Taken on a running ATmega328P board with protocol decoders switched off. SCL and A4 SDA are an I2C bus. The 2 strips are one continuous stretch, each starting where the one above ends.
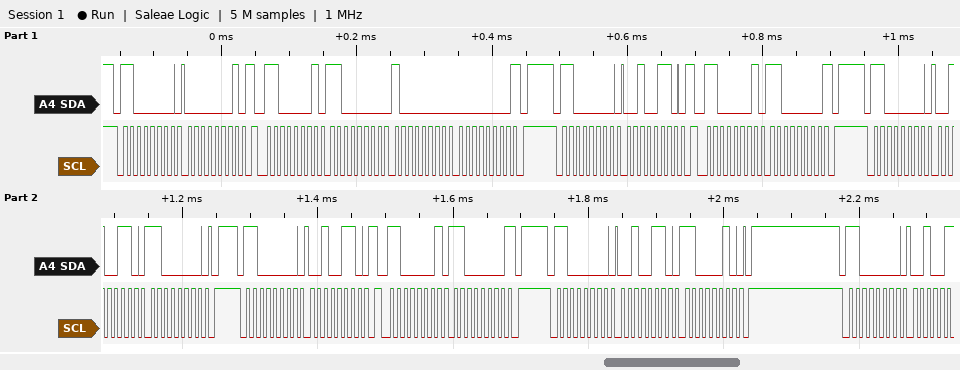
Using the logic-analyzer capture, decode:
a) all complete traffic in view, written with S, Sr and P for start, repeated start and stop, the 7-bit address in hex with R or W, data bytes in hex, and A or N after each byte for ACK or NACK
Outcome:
S 60W A 01 A Sr 60R A C0 A 80 A 00 N P S 60W A 26 A Sr 60R A C0 N P S 60W A 26 A C0 A P S 60W A 26 A Sr 60R A C0 N P S 60W A 26 A C2 A P S 60W A
